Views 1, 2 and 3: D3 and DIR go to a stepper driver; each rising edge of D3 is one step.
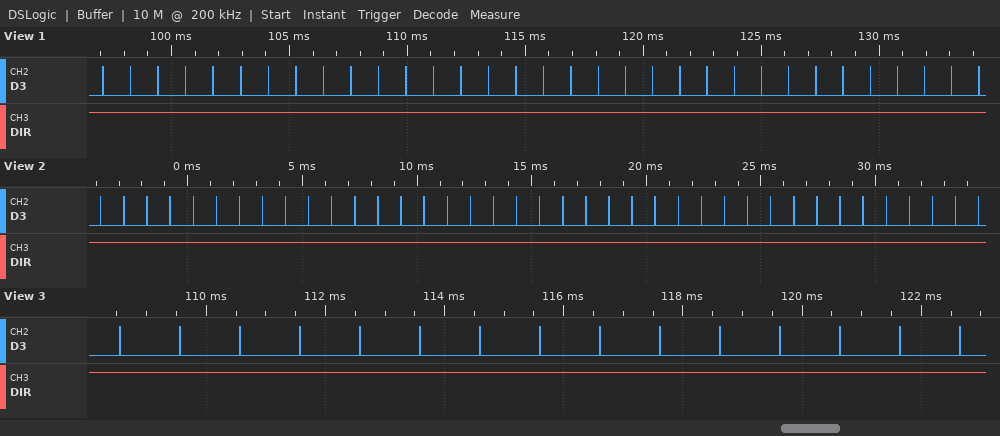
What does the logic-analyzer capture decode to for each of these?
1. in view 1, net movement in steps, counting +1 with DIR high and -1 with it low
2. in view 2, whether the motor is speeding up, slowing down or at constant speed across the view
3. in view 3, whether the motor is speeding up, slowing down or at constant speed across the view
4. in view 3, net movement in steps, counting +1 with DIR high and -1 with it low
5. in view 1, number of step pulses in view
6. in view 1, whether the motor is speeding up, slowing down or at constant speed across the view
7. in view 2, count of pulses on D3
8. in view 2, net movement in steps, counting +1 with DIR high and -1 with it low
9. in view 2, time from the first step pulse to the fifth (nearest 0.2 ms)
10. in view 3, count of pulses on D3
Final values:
+33
constant speed
constant speed
+15
33
constant speed
39
+39
4.0 ms
15
